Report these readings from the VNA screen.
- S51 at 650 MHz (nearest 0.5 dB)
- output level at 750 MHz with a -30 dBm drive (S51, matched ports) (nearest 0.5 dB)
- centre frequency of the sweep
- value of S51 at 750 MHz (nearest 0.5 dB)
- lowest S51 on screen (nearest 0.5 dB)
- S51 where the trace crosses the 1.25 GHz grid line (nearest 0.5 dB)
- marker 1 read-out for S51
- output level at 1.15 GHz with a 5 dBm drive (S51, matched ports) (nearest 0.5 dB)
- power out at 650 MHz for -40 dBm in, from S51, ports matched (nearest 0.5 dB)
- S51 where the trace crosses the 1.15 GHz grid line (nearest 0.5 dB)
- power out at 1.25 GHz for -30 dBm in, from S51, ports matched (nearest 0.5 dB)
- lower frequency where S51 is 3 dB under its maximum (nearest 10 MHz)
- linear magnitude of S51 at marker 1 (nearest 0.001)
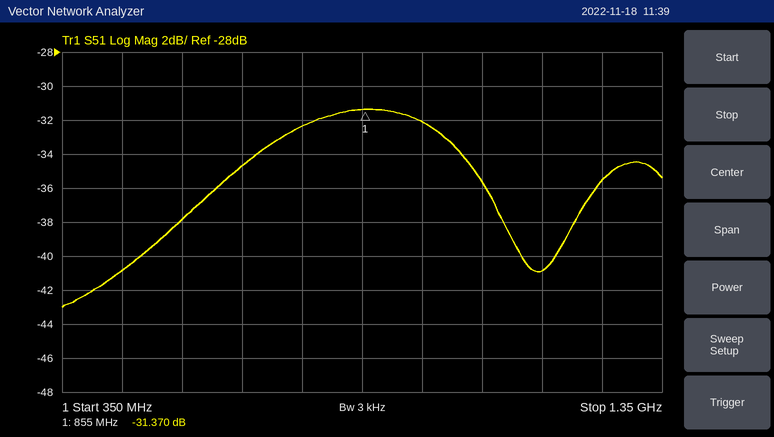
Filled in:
-34.5 dB
-62.5 dBm
850 MHz
-32.5 dB
-43.0 dB
-35.5 dB
-31.370 dB
-36.0 dBm
-74.5 dBm
-41.0 dB
-65.5 dBm
660 MHz
0.027
